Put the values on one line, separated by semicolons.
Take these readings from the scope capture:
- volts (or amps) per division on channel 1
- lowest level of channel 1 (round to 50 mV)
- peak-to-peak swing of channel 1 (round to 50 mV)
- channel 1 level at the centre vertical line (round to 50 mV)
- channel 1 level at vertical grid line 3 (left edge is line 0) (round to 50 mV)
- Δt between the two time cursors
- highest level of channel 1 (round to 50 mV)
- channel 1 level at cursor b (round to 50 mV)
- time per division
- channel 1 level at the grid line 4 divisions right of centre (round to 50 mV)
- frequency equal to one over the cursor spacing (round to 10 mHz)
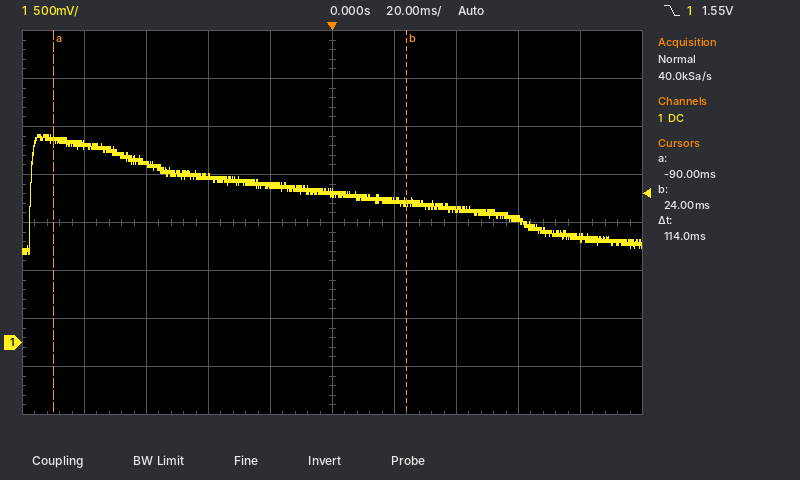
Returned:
500 mV; 900 mV; 1.25 V; 1.55 V; 1.75 V; 114 ms; 2.15 V; 1.45 V; 20 ms; 1.10 V; 8.77 Hz
